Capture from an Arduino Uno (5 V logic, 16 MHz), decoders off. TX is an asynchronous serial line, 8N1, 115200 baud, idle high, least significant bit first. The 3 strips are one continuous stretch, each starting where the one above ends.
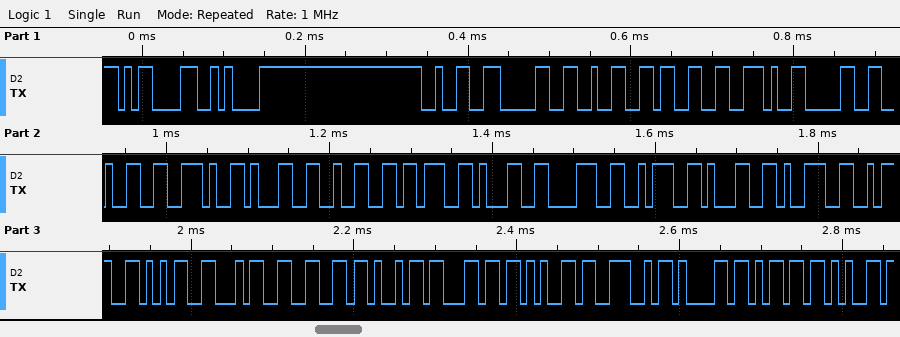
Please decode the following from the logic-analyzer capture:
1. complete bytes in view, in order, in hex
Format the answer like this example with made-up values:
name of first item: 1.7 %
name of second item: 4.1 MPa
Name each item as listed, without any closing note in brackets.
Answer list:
complete bytes in view, in order, in hex: 0D 0A 32 30 32 33 2E 30 32 2E 31 32 3B 31 38 3A 31 39 3A 35 34 66 69 6C 65 4E 61 6D 65
